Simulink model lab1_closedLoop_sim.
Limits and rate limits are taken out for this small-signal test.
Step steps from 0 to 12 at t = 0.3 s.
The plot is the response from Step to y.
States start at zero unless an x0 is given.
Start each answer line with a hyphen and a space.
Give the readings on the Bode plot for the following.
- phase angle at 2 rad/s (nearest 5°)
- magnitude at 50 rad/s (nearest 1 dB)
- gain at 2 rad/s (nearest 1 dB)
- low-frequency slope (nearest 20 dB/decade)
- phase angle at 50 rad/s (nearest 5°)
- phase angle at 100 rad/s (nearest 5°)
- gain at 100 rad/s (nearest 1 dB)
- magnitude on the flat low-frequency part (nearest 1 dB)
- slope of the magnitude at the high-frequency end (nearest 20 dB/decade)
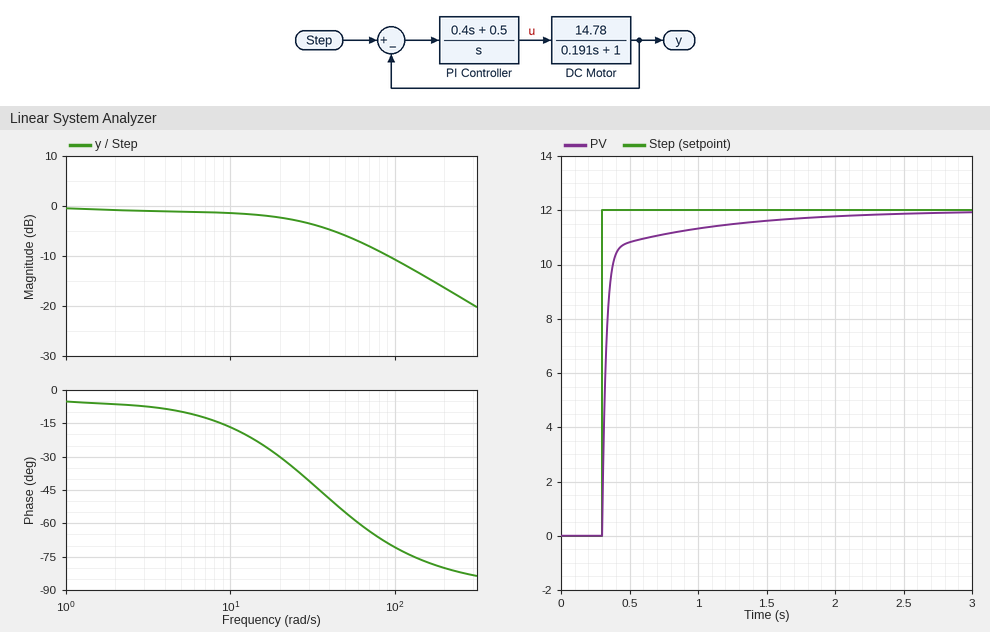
- -5°
- -6 dB
- -1 dB
- 0 dB/decade
- -55°
- -70°
- -11 dB
- -1 dB
- -20 dB/decade
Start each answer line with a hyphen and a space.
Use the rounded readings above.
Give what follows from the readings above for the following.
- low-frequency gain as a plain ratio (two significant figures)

- 0.89
